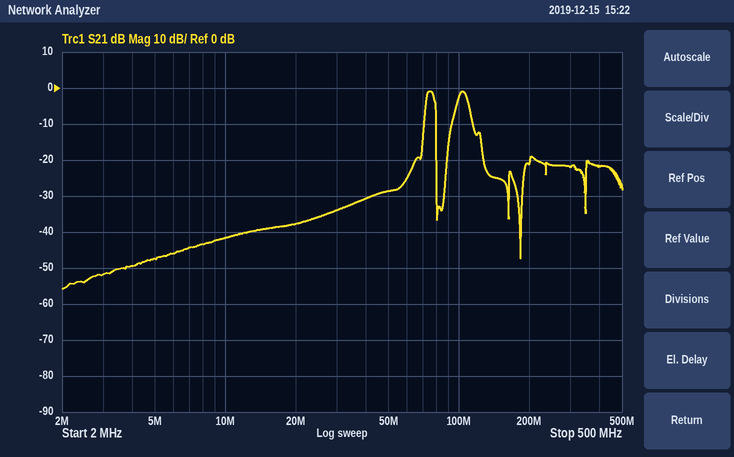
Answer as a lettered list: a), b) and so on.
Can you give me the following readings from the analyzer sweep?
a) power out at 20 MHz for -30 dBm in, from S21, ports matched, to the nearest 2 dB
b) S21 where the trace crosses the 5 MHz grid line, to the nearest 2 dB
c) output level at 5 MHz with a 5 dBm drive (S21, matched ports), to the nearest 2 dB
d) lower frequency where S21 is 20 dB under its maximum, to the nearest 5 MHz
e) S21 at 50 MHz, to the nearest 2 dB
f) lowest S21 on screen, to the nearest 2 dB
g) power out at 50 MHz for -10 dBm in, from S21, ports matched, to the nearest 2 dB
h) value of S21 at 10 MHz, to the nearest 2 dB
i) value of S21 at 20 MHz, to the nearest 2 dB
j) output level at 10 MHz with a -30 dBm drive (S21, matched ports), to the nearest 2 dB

a) -68 dBm
b) -48 dB
c) -42 dBm
d) 65 MHz
e) -28 dB
f) -56 dB
g) -38 dBm
h) -42 dB
i) -38 dB
j) -72 dBm
